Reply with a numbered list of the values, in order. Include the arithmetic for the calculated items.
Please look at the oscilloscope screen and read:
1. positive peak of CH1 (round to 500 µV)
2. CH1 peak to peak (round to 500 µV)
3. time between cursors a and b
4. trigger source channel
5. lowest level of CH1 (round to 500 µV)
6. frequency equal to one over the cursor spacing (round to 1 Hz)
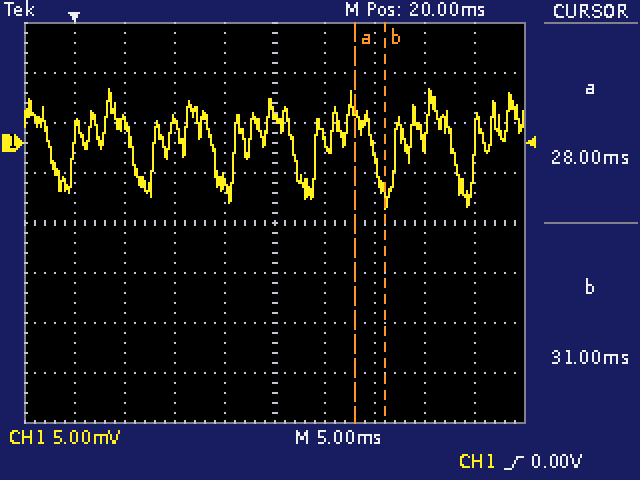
1. 5.5 mV
2. 5.5 mV − (-6.5 mV) = 12.0 mV
3. 31 ms − (28 ms) = 3.0 ms
4. CH1
5. -6.5 mV
6. 1 / 3.0 ms ≈ 333 Hz
